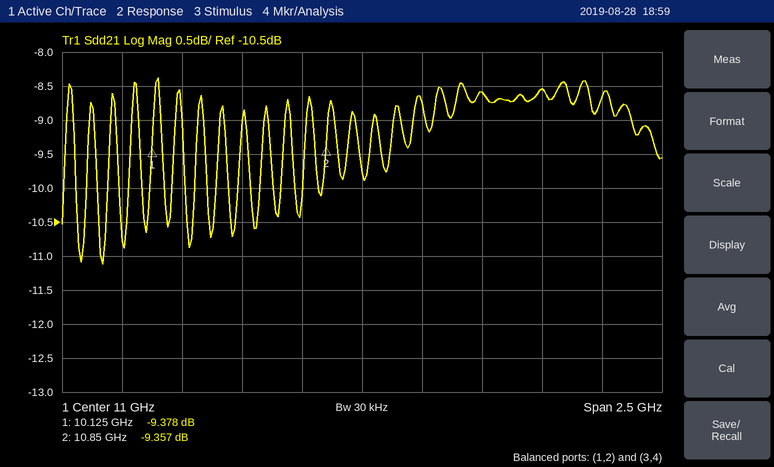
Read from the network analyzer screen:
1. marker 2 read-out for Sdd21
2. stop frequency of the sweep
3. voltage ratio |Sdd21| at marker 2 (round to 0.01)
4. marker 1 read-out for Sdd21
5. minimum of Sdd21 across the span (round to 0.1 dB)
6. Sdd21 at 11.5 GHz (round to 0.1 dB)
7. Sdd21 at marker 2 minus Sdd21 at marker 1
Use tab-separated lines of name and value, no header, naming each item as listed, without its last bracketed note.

marker 2 read-out for Sdd21	-9.357 dB
stop frequency of the sweep	12.25 GHz
voltage ratio |Sdd21| at marker 2	0.34
marker 1 read-out for Sdd21	-9.378 dB
minimum of Sdd21 across the span	-11.1 dB
Sdd21 at 11.5 GHz	-8.6 dB
Sdd21 at marker 2 minus Sdd21 at marker 1	0.021 dB
